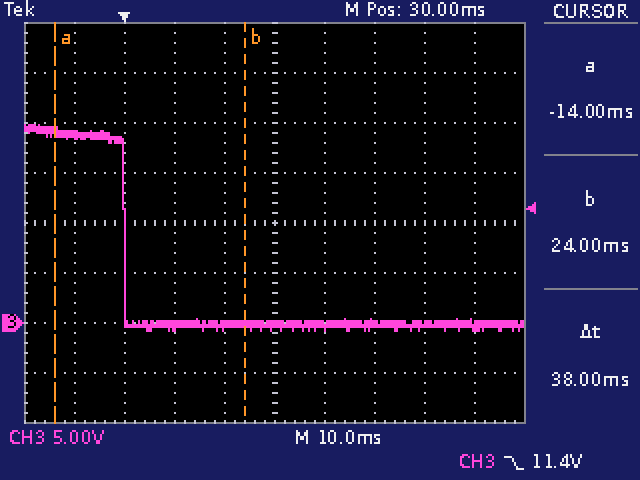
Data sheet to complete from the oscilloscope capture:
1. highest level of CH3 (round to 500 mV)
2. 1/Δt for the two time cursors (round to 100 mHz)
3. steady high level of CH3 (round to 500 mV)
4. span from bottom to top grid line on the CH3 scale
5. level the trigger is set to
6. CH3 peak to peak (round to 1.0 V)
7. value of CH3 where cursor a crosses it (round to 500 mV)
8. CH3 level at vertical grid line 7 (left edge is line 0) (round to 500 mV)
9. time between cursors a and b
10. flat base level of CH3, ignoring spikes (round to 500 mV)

20.0 V
26.3 Hz
19.0 V
40 V
11.4 V
21.0 V
19.0 V
0.0 V
38 ms
0.0 V
